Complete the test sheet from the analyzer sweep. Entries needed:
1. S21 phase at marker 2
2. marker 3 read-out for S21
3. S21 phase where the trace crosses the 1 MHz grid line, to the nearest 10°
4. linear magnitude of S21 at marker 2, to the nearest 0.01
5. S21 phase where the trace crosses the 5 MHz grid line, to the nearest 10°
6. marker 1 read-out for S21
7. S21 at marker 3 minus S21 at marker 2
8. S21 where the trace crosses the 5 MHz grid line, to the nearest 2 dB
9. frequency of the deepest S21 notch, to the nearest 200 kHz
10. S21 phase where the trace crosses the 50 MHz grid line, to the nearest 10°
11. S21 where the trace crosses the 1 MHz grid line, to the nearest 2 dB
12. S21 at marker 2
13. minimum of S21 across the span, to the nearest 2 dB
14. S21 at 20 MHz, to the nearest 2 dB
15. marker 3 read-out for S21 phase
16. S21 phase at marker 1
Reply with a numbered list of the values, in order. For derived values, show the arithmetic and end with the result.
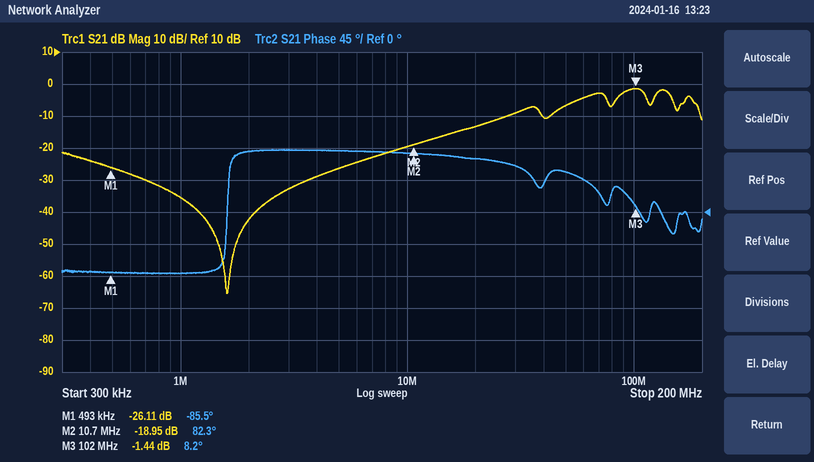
1. 82.3°
2. -1.44 dB
3. -90°
4. 10^(-18.95/20) ≈ 0.11
5. 90°
6. -26.11 dB
7. -1.44 − (-18.95) = 17.51 dB
8. -26 dB
9. 1.6 MHz
10. 60°
11. -36 dB
12. -18.95 dB
13. -66 dB
14. -14 dB
15. 8.2°
16. -85.5°
